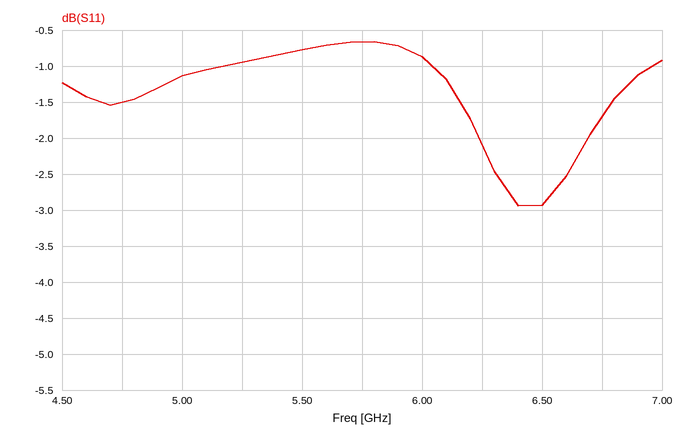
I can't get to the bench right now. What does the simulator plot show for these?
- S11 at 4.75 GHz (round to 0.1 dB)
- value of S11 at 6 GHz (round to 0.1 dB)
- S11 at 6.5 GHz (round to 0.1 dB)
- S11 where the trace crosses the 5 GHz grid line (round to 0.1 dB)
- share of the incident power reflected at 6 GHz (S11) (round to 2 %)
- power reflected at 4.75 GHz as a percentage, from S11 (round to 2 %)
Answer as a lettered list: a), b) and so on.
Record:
a) -1.5 dB
b) -0.9 dB
c) -2.9 dB
d) -1.1 dB
e) 82 %
f) 70 %
